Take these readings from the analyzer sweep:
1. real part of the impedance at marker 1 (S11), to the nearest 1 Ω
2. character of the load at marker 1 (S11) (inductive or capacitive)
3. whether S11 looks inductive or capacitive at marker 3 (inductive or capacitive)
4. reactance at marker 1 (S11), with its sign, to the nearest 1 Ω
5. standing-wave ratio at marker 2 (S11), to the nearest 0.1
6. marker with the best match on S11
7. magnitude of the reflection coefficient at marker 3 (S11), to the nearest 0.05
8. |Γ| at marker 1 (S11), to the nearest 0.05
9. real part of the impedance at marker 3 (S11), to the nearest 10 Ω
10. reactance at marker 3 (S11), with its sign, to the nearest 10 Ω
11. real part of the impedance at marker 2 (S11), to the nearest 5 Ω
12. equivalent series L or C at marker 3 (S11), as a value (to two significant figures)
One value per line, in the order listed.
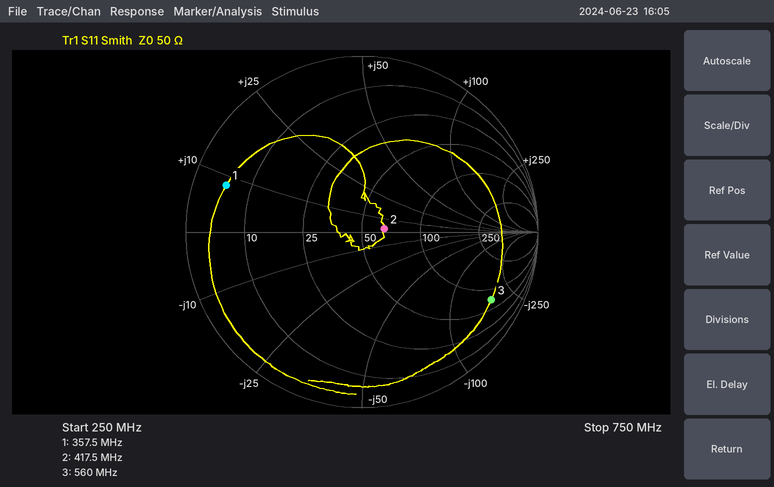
5 Ω
inductive
capacitive
+8 Ω
1.3
marker 2
0.85
0.80
70 Ω
-180 Ω
65 Ω
1.6 pF
